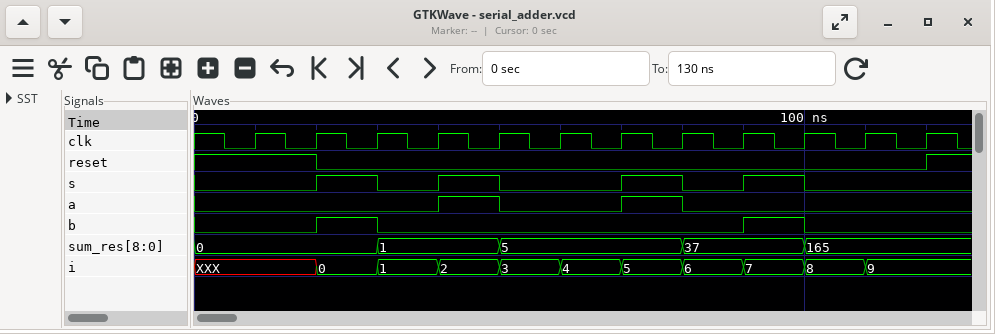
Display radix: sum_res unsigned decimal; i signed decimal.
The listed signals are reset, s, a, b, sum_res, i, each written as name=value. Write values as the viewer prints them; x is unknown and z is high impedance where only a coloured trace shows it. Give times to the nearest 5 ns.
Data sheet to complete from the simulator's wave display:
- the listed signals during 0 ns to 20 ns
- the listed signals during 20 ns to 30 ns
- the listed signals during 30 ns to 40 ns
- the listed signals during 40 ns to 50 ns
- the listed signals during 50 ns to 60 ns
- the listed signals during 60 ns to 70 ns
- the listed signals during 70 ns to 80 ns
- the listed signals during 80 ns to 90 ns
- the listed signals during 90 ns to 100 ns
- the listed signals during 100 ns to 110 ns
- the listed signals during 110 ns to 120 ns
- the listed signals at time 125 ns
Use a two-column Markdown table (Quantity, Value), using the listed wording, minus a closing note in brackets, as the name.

| Quantity | Value |
|---|---|
| the listed signals during 0 ns to 20 ns | reset=1, s=0, a=0, b=0, sum_res=0, i=XXX |
| the listed signals during 20 ns to 30 ns | reset=0, s=1, a=0, b=1, sum_res=0, i=0 |
| the listed signals during 30 ns to 40 ns | reset=0, s=0, a=0, b=0, sum_res=1, i=1 |
| the listed signals during 40 ns to 50 ns | reset=0, s=1, a=1, b=0, sum_res=1, i=2 |
| the listed signals during 50 ns to 60 ns | reset=0, s=0, a=0, b=0, sum_res=5, i=3 |
| the listed signals during 60 ns to 70 ns | reset=0, s=0, a=0, b=0, sum_res=5, i=4 |
| the listed signals during 70 ns to 80 ns | reset=0, s=1, a=1, b=0, sum_res=5, i=5 |
| the listed signals during 80 ns to 90 ns | reset=0, s=0, a=0, b=0, sum_res=37, i=6 |
| the listed signals during 90 ns to 100 ns | reset=0, s=1, a=0, b=1, sum_res=37, i=7 |
| the listed signals during 100 ns to 110 ns | reset=0, s=0, a=0, b=0, sum_res=165, i=8 |
| the listed signals during 110 ns to 120 ns | reset=0, s=0, a=0, b=0, sum_res=165, i=9 |
| the listed signals at time 125 ns | reset=1, s=0, a=0, b=0, sum_res=165, i=9 |
